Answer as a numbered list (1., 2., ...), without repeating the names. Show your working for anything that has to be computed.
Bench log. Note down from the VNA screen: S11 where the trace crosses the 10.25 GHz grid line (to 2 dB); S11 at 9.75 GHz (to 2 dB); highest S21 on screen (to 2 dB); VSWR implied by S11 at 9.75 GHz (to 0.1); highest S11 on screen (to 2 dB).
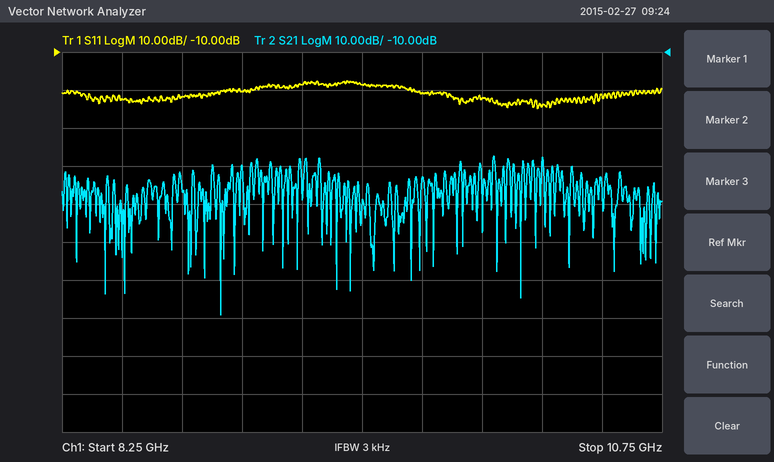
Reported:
1. -24 dB
2. -20 dB
3. -38 dB
4. |Γ| = 10^(-20/20) = 0.1000; VSWR = (1 + 0.1000)/(1 − 0.1000) ≈ 1.2
5. -18 dB
